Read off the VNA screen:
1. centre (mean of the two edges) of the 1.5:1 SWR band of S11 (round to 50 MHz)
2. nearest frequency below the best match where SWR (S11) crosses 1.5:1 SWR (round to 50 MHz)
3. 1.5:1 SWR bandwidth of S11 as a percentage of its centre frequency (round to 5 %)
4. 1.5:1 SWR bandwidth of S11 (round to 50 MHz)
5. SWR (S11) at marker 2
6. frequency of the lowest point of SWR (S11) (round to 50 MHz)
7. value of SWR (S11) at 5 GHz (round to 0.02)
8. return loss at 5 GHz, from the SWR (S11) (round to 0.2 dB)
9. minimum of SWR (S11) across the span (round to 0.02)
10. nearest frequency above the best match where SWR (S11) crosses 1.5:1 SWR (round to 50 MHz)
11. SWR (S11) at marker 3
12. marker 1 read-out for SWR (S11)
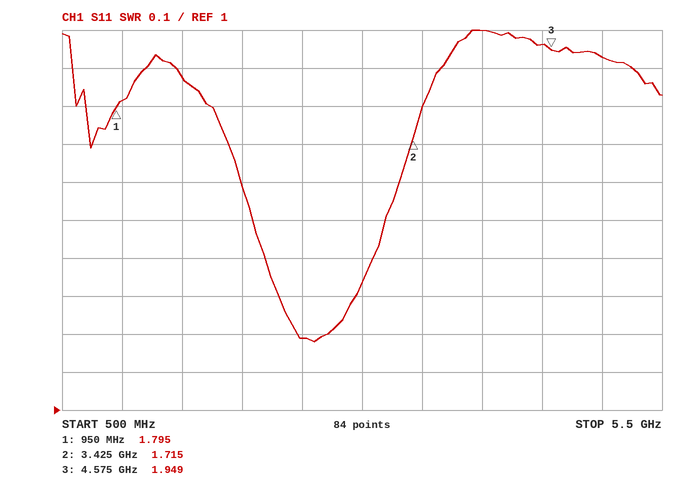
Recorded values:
2.65 GHz
2.10 GHz
40 %
1.10 GHz
1.715
2.60 GHz
1.92
10.0 dB
1.18
3.20 GHz
1.949
1.795
